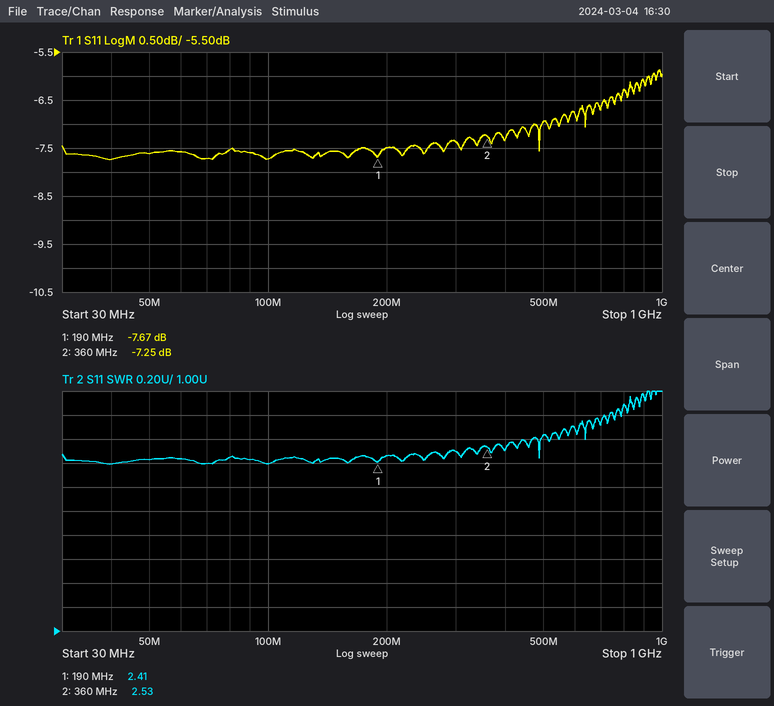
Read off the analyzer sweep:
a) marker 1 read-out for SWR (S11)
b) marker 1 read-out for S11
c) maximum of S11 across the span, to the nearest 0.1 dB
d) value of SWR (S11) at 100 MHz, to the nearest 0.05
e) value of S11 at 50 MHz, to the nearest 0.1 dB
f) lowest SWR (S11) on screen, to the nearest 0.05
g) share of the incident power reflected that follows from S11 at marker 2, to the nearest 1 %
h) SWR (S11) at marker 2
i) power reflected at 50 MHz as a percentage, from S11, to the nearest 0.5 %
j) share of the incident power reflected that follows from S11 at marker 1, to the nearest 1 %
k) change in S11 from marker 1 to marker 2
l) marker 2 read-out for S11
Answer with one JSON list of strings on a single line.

["2.41", "-7.67 dB", "-5.9 dB", "2.40", "-7.6 dB", "2.40", "19 %", "2.53", "17.5 %", "17 %", "0.42 dB", "-7.25 dB"]
